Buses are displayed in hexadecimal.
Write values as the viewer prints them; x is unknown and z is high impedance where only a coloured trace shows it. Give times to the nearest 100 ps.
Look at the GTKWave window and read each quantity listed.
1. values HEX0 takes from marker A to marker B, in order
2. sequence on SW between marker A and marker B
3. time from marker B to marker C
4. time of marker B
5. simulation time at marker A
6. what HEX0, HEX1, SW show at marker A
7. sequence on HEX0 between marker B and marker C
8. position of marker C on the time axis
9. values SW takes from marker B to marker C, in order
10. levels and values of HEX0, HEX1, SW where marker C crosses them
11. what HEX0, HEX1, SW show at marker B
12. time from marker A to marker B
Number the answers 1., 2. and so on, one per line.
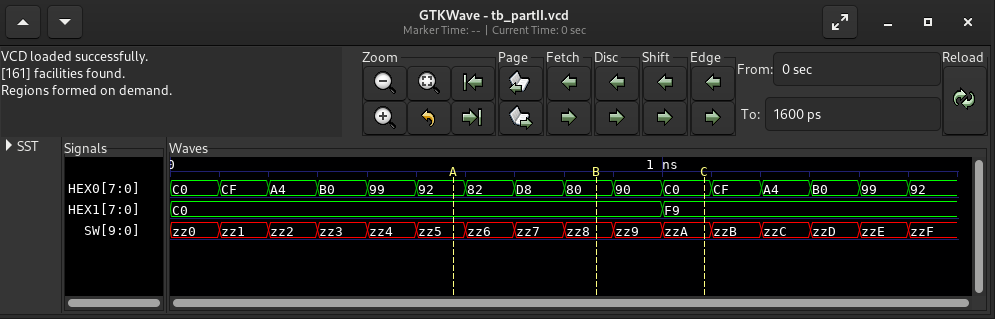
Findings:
1. 92, 82, D8, 80
2. zz5, zz6, zz7, zz8
3. 200 ps
4. 900 ps
5. 600 ps
6. HEX0=92, HEX1=C0, SW=zz5
7. 80, 90, C0
8. 1100 ps
9. zz8, zz9, zzA
10. HEX0=C0, HEX1=F9, SW=zzA
11. HEX0=80, HEX1=C0, SW=zz8
12. 300 ps
